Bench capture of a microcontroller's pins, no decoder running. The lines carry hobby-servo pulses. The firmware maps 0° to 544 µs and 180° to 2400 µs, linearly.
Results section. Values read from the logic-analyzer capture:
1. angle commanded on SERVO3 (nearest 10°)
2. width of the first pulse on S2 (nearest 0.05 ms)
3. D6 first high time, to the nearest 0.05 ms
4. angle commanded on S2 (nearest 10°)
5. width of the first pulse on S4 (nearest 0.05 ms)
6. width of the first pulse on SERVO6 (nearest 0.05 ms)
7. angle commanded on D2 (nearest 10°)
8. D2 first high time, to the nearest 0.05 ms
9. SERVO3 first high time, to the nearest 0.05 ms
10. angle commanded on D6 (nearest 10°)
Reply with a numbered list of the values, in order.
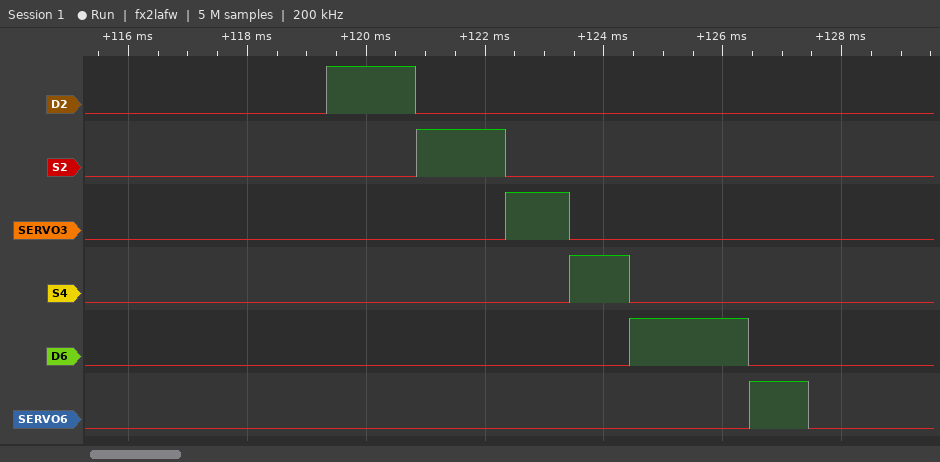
1. 50°
2. 1.50 ms
3. 2.00 ms
4. 90°
5. 1.00 ms
6. 1.00 ms
7. 90°
8. 1.50 ms
9. 1.05 ms
10. 140°
